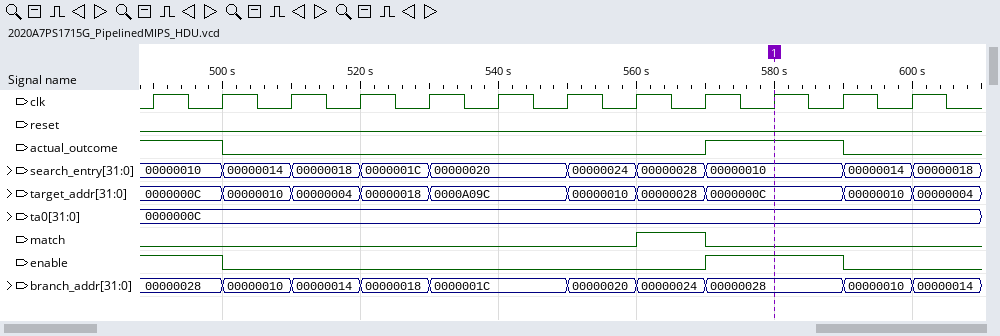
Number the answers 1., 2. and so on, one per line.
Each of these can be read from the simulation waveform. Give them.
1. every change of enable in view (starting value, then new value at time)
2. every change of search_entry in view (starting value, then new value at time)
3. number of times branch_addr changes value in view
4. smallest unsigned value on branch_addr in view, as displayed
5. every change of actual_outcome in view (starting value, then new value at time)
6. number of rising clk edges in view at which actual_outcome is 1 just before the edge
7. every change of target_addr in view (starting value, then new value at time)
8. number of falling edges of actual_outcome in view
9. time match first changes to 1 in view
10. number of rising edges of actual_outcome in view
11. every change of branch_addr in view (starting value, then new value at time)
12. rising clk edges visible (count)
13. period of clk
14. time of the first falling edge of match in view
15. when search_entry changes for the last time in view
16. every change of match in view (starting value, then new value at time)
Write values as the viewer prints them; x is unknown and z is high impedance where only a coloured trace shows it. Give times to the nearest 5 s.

1. 1, 0 at 500 s, 1 at 570 s, 0 at 590 s
2. 00000010, 00000014 at 500 s, 00000018 at 510 s, 0000001C at 520 s, 00000020 at 530 s, 00000024 at 550 s, 00000028 at 560 s, 00000010 at 570 s, 00000014 at 590 s, 00000018 at 600 s
3. 9
4. 00000010
5. 1, 0 at 500 s, 1 at 570 s, 0 at 590 s
6. 4
7. 0000000C, 00000010 at 500 s, 00000004 at 510 s, 00000018 at 520 s, 0000A09C at 530 s, 00000010 at 550 s, 00000028 at 560 s, 0000000C at 570 s, 00000010 at 590 s, 00000004 at 600 s
8. 2
9. 560 s
10. 1
11. 00000028, 00000010 at 500 s, 00000014 at 510 s, 00000018 at 520 s, 0000001C at 530 s, 00000020 at 550 s, 00000024 at 560 s, 00000028 at 570 s, 00000010 at 590 s, 00000014 at 600 s
12. 12
13. 10 s
14. 570 s
15. 600 s
16. 0, 1 at 560 s, 0 at 570 s
